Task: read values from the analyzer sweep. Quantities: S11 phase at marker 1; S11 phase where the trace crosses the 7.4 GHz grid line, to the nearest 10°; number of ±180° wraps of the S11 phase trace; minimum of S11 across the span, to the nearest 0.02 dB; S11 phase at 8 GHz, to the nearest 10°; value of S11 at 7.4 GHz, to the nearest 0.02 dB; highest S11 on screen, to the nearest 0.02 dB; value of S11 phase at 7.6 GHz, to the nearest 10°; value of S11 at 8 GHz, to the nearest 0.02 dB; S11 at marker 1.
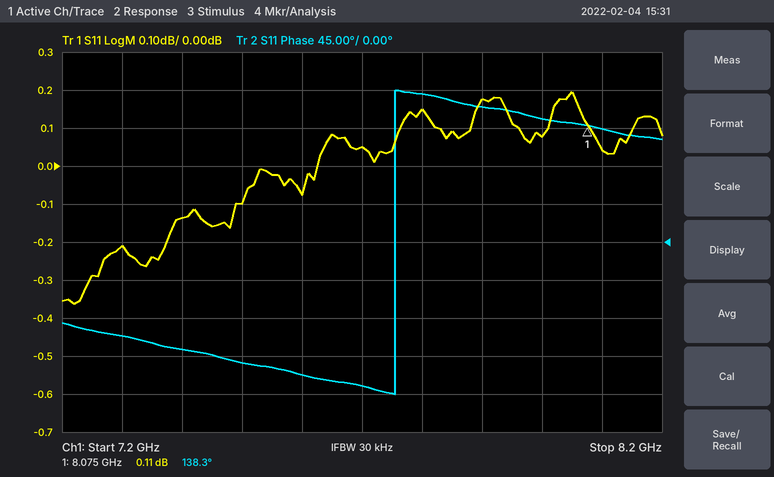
138.3°
-130°
1
-0.36 dB
150°
-0.14 dB
0.20 dB
-160°
0.08 dB
0.11 dB
